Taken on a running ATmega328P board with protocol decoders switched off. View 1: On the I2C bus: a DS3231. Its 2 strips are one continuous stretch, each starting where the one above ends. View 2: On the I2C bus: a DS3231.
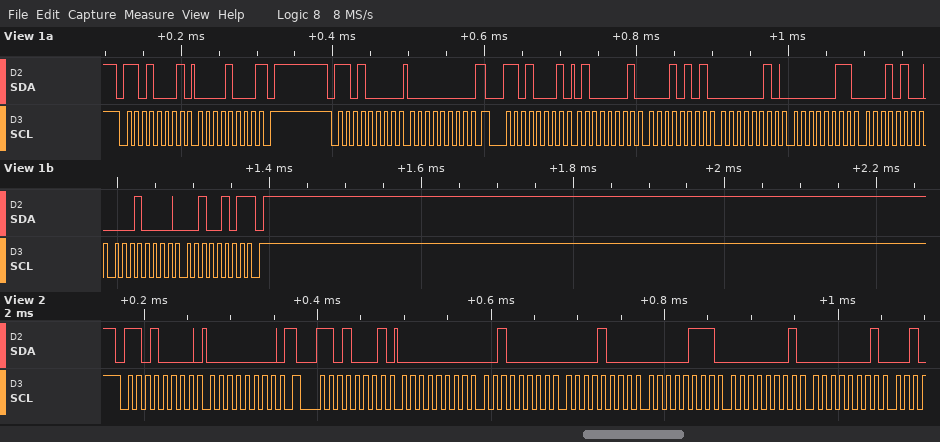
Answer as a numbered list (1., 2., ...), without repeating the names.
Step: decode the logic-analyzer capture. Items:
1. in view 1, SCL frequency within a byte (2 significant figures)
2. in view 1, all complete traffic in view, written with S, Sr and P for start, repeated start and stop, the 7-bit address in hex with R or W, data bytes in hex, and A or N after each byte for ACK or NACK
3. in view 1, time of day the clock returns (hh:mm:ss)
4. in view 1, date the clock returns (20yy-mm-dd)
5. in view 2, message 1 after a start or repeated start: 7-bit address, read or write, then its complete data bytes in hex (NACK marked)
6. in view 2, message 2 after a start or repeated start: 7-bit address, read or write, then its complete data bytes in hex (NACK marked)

1. 100 kHz
2. S 68R A 08 N P S 68W A 00 A Sr 68R A 41 A 15 A 02 A 03 A 14 A 10 A 25 N P
3. 02:15:41
4. 2025-10-14
5. 0x68 write: 00
6. 0x68 read: 00 20 08 07 01 01
